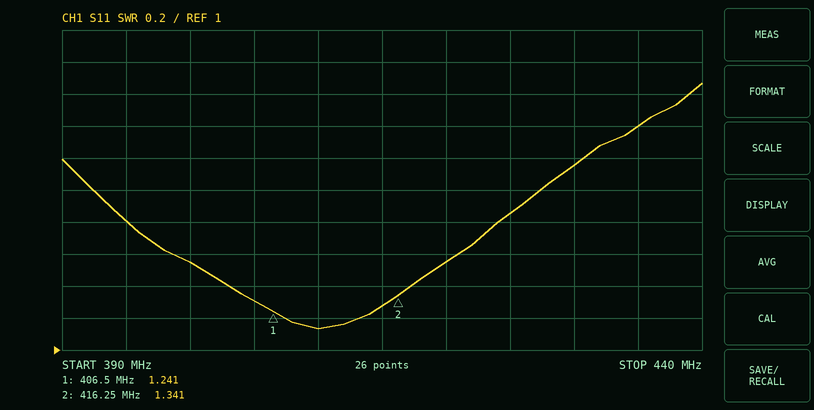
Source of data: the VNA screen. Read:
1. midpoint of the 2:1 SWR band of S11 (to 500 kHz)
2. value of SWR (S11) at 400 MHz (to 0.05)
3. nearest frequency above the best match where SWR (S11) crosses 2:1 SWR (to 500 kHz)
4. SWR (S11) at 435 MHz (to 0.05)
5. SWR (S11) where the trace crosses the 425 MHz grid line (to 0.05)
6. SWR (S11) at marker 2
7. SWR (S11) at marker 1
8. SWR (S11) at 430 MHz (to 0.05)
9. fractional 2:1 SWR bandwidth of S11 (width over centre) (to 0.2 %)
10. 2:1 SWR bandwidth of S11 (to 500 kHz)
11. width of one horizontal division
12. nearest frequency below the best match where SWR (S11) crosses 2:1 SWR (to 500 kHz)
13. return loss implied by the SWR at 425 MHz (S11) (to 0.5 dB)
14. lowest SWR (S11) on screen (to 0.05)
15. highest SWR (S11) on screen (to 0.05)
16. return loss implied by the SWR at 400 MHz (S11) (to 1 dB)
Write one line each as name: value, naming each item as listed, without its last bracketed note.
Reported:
midpoint of the 2:1 SWR band of S11: 410.0 MHz
value of SWR (S11) at 400 MHz: 1.55
nearest frequency above the best match where SWR (S11) crosses 2:1 SWR: 427.5 MHz
SWR (S11) at 435 MHz: 2.40
SWR (S11) where the trace crosses the 425 MHz grid line: 1.85
SWR (S11) at marker 2: 1.341
SWR (S11) at marker 1: 1.241
SWR (S11) at 430 MHz: 2.15
fractional 2:1 SWR bandwidth of S11 (width over centre): 8.6 %
2:1 SWR bandwidth of S11: 35.0 MHz
width of one horizontal division: 5 MHz
nearest frequency below the best match where SWR (S11) crosses 2:1 SWR: 392.5 MHz
return loss implied by the SWR at 425 MHz (S11): 10.5 dB
lowest SWR (S11) on screen: 1.15
highest SWR (S11) on screen: 2.65
return loss implied by the SWR at 400 MHz (S11): 13 dB
